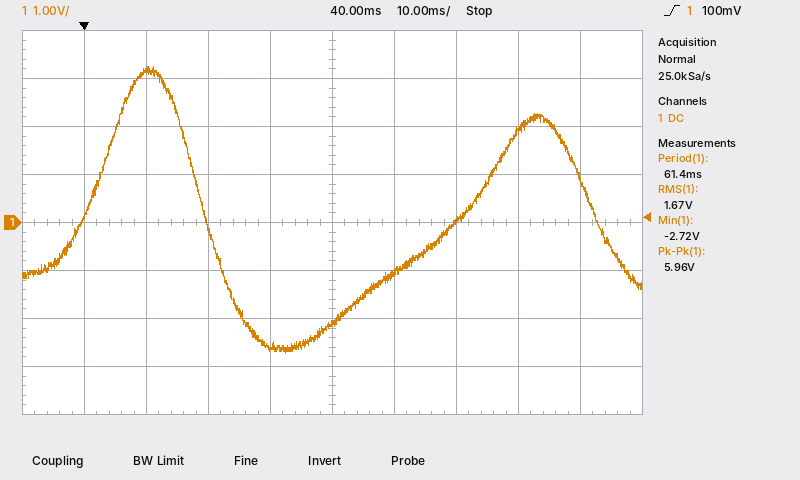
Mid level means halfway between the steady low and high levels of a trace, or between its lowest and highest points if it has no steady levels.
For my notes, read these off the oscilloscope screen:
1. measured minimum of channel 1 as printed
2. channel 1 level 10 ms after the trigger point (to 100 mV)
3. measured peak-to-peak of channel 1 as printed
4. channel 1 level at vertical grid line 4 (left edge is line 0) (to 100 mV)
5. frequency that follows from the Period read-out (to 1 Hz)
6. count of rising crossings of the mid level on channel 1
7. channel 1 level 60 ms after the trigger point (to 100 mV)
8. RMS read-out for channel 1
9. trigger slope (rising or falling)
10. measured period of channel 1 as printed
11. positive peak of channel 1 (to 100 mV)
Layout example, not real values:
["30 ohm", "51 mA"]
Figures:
["-2.72 V", "3.2 V", "5.96 V", "-2.6 V", "16 Hz", "2", "0.0 V", "1.67 V", "rising", "61.4 ms", "3.2 V"]
